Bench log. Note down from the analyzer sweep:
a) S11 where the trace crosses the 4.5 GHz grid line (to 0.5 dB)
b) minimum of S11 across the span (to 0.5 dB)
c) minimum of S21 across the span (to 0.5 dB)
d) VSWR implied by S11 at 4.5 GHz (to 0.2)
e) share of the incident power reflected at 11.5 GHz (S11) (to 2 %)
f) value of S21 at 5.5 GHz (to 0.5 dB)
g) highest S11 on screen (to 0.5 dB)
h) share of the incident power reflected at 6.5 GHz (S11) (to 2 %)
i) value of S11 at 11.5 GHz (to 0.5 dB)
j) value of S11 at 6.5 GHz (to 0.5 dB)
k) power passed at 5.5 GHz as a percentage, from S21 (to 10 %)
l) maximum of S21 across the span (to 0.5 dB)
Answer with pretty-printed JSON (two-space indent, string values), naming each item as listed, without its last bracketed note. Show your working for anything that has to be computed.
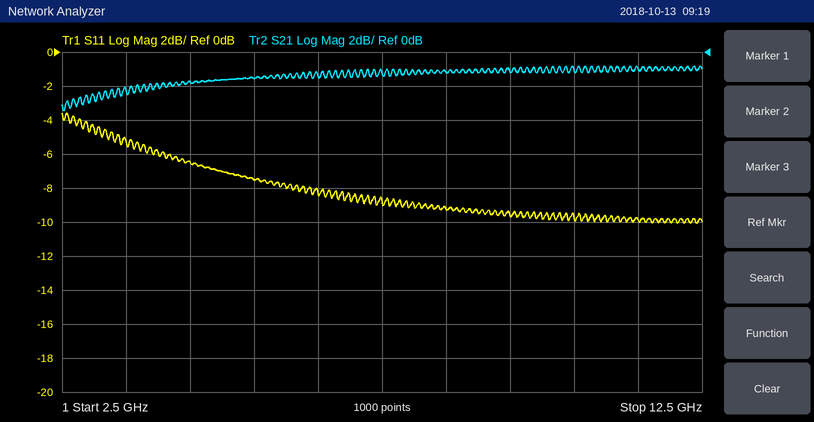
{
  "S11 where the trace crosses the 4.5 GHz grid line": "-6.5 dB",
  "minimum of S11 across the span": "-10.0 dB",
  "minimum of S21 across the span": "-3.5 dB",
  "VSWR implied by S11 at 4.5 GHz": "|Γ| = 10^(-6.5/20) = 0.4732; VSWR = (1 + 0.4732)/(1 − 0.4732) ≈ 2.8",
  "share of the incident power reflected at 11.5 GHz (S11)": "10^(-10/10) ≈ 10 %",
  "value of S21 at 5.5 GHz": "-1.5 dB",
  "highest S11 on screen": "-3.5 dB",
  "share of the incident power reflected at 6.5 GHz (S11)": "10^(-8.5/10) ≈ 14 %",
  "value of S11 at 11.5 GHz": "-10.0 dB",
  "value of S11 at 6.5 GHz": "-8.5 dB",
  "power passed at 5.5 GHz as a percentage, from S21": "10^(-1.5/10) ≈ 70.8 %, so 70 % to the nearest 10 %",
  "maximum of S21 across the span": "-1.0 dB"
}
